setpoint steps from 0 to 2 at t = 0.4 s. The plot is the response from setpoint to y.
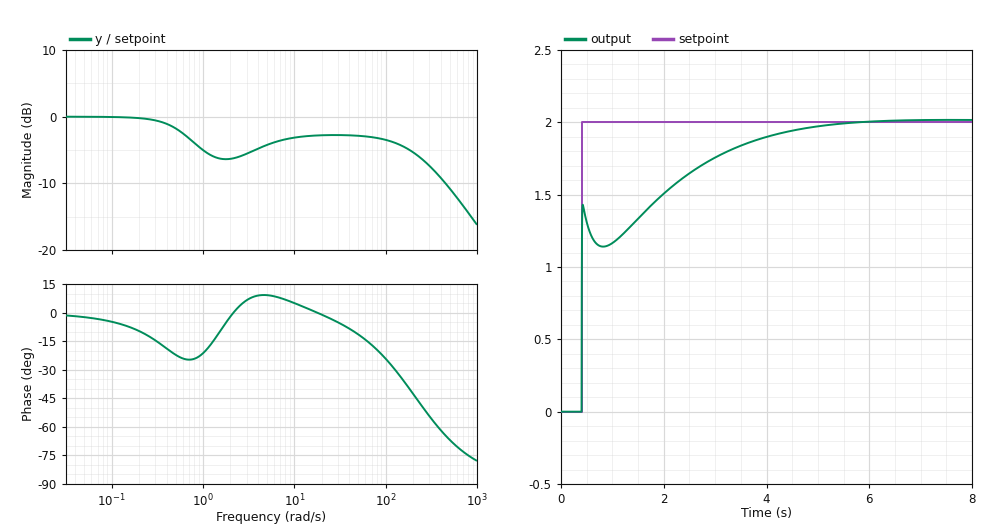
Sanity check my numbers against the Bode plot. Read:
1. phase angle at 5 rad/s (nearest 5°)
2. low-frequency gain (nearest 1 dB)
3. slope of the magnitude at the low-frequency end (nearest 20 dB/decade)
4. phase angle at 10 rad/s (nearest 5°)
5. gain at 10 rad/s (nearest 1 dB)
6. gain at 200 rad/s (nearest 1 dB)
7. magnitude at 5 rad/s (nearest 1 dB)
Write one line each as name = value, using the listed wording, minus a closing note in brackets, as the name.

phase angle at 5 rad/s = 10°
low-frequency gain = 0 dB
slope of the magnitude at the low-frequency end = 0 dB/decade
phase angle at 10 rad/s = 5°
gain at 10 rad/s = -3 dB
gain at 200 rad/s = -5 dB
magnitude at 5 rad/s = -4 dB
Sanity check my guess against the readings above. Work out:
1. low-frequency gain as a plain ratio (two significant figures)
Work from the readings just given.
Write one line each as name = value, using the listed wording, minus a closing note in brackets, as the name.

low-frequency gain as a plain ratio = 1.0
